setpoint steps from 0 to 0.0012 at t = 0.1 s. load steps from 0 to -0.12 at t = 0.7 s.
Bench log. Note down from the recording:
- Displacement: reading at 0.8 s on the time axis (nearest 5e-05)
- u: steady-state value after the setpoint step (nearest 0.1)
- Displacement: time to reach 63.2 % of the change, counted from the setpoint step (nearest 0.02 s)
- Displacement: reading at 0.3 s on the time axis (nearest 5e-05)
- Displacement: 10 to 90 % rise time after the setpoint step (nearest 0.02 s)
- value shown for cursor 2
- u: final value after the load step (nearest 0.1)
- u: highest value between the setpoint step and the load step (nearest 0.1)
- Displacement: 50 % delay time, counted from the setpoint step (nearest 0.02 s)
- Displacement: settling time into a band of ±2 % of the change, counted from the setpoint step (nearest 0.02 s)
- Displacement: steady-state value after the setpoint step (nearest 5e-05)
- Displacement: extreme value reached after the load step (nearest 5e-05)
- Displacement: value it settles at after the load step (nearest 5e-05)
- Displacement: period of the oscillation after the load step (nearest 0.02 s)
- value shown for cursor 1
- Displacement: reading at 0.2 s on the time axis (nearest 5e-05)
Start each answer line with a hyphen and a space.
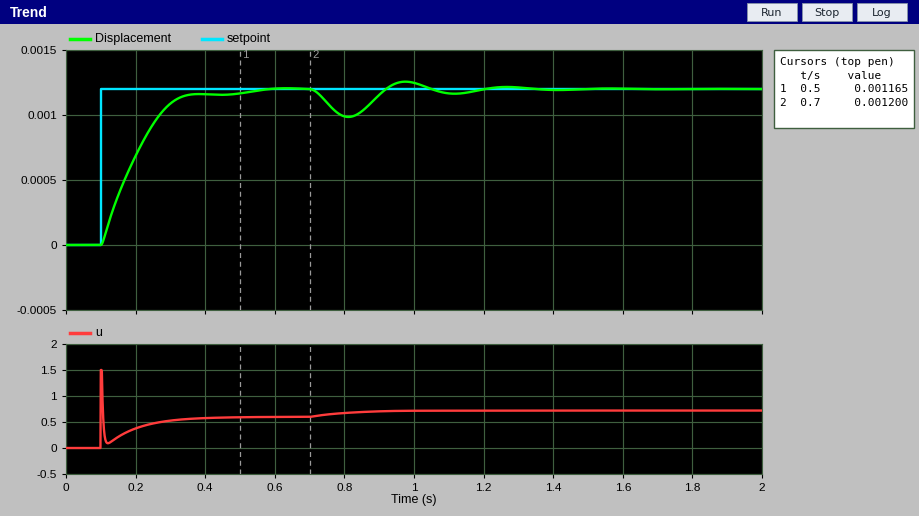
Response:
- 0.00100
- 0.6
- 0.12 s
- 0.00110
- 0.18 s
- 0.001200
- 0.7
- 1.5
- 0.08 s
- 0.42 s
- 0.00120
- 0.00100
- 0.00120
- 0.30 s
- 0.001165
- 0.00070
